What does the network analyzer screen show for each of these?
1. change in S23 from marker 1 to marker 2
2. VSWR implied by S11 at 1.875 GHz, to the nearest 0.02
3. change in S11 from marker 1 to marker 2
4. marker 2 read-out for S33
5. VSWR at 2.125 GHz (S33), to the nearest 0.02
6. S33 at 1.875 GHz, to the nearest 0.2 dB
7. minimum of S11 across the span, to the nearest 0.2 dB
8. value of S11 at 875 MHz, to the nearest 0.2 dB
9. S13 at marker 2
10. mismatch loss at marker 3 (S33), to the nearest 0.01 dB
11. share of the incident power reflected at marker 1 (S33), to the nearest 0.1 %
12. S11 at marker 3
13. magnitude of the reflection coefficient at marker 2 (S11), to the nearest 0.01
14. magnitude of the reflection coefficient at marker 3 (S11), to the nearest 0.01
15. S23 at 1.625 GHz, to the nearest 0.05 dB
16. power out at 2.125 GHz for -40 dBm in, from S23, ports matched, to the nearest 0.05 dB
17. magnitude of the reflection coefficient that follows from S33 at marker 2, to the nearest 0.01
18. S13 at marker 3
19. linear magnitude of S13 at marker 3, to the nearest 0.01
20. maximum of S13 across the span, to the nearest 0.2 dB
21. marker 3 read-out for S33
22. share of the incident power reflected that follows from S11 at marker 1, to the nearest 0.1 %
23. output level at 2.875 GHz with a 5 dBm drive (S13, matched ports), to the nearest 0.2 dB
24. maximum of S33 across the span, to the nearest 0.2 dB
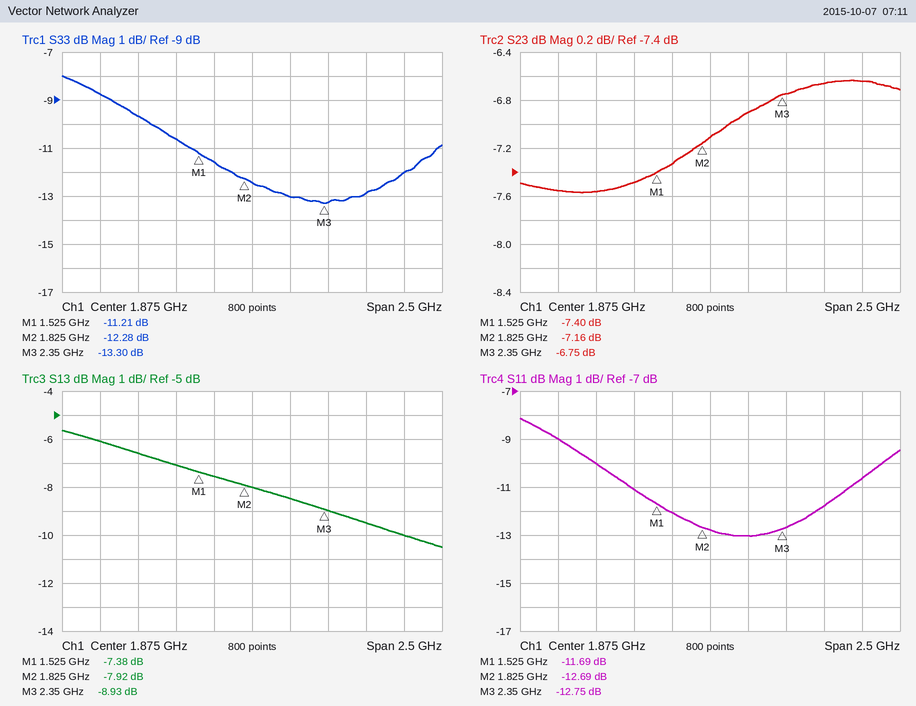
0.24 dB
1.60
-1.00 dB
-12.28 dB
1.58
-12.4 dB
-13.0 dB
-9.0 dB
-7.92 dB
0.21 dB
7.6 %
-12.75 dB
0.23
0.23
-7.35 dB
-46.90 dBm
0.24
-8.93 dB
0.36
-5.6 dB
-13.30 dB
6.8 %
-5.0 dBm
-8.0 dB
